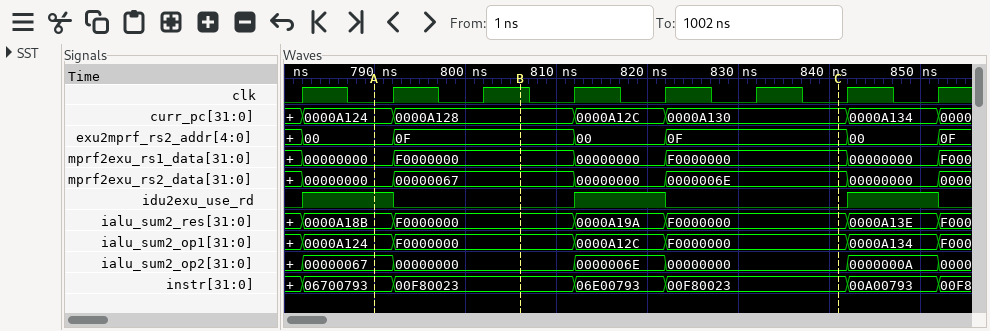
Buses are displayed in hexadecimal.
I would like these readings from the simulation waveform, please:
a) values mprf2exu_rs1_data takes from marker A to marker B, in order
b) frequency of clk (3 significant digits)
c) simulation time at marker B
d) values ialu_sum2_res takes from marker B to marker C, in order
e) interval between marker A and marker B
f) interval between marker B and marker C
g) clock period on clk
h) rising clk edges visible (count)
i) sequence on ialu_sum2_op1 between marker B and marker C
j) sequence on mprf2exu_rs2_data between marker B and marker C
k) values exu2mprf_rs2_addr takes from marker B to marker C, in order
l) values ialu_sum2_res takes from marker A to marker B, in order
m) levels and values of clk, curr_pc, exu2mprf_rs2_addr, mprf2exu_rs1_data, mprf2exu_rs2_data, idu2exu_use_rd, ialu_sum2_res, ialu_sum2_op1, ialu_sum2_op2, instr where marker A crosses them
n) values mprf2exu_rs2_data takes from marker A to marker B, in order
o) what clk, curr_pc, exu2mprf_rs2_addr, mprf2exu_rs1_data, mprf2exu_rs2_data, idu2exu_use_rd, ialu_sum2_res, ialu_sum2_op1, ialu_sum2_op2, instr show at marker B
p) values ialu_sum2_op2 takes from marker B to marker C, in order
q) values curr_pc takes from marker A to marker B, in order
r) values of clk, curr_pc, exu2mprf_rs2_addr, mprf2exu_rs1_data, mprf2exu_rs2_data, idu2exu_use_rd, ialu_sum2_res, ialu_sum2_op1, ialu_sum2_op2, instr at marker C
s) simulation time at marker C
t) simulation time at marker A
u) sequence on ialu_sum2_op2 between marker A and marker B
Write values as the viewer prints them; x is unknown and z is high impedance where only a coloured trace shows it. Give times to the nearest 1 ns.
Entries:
00000000, F0000000
100 MHz
806 ns
F0000000, 0000A19A, F0000000
16 ns
35 ns
10 ns
8
F0000000, 0000A12C, F0000000
00000067, 00000000, 0000006E
0F, 00, 0F
0000A18B, F0000000
clk=0, curr_pc=0000A124, exu2mprf_rs2_addr=00, mprf2exu_rs1_data=00000000, mprf2exu_rs2_data=00000000, idu2exu_use_rd=1, ialu_sum2_res=0000A18B, ialu_sum2_op1=0000A124, ialu_sum2_op2=00000067, instr=06700793
00000000, 00000067
clk=1, curr_pc=0000A128, exu2mprf_rs2_addr=0F, mprf2exu_rs1_data=F0000000, mprf2exu_rs2_data=00000067, idu2exu_use_rd=0, ialu_sum2_res=F0000000, ialu_sum2_op1=F0000000, ialu_sum2_op2=00000000, instr=00F80023
00000000, 0000006E, 00000000
0000A124, 0000A128
clk=0, curr_pc=0000A130, exu2mprf_rs2_addr=0F, mprf2exu_rs1_data=F0000000, mprf2exu_rs2_data=0000006E, idu2exu_use_rd=0, ialu_sum2_res=F0000000, ialu_sum2_op1=F0000000, ialu_sum2_op2=00000000, instr=00F80023
841 ns
790 ns
00000067, 00000000
